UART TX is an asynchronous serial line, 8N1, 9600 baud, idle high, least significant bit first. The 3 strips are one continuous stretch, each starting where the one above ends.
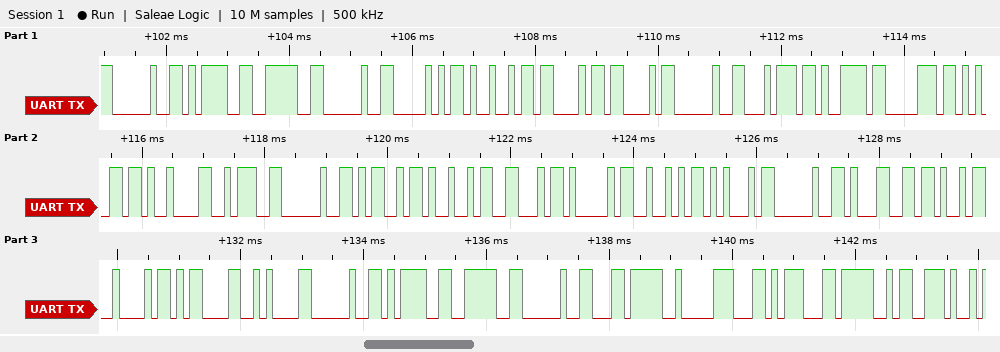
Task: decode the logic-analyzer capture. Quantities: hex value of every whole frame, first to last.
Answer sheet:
20 3D 3E 20 50 49 43 43 20 74 79 70 65 09 3A 20 4D 49 46 41 52 45 20 31 4B 42 0D 0A 20 3D 3E 20 EC 82 AC EC 9A
